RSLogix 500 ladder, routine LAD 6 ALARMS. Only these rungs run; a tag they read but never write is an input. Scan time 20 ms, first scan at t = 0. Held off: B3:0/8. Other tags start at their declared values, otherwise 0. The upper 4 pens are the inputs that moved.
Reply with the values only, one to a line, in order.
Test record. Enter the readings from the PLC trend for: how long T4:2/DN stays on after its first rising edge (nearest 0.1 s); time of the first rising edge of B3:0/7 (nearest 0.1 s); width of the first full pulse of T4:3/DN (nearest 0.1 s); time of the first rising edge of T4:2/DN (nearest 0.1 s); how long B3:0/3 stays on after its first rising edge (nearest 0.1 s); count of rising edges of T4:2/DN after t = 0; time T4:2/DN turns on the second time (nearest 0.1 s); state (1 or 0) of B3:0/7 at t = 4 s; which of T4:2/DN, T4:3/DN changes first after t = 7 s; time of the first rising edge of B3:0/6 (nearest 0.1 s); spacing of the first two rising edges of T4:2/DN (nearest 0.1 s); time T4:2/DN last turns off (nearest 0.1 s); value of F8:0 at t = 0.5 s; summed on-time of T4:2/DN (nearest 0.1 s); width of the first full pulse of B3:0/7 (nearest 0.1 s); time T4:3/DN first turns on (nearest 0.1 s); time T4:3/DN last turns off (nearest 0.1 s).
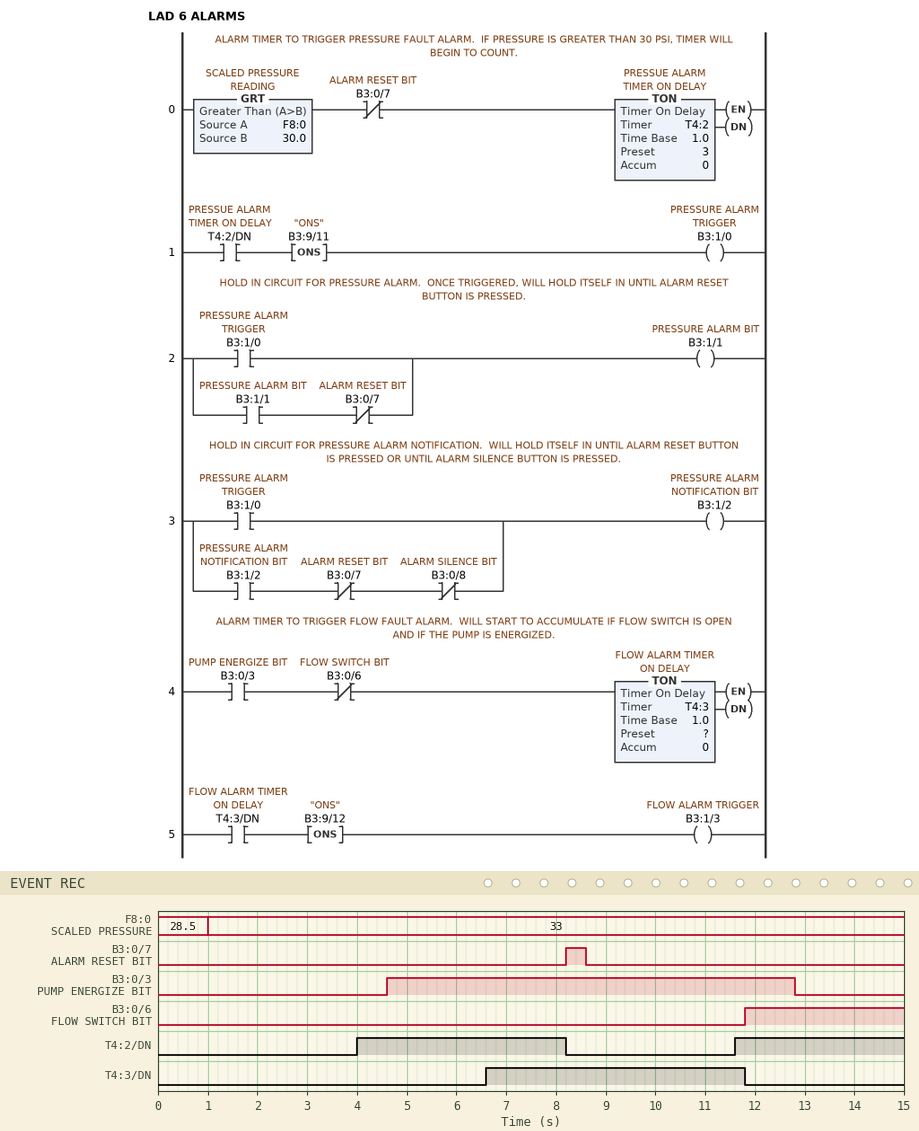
4.2 s
8.2 s
5.2 s
4.0 s
8.2 s
2
11.6 s
0
T4:2/DN
11.8 s
7.6 s
8.2 s
28.5
7.6 s
0.4 s
6.6 s
11.8 s
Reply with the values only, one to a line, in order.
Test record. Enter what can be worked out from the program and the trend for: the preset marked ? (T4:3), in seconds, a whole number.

2 s
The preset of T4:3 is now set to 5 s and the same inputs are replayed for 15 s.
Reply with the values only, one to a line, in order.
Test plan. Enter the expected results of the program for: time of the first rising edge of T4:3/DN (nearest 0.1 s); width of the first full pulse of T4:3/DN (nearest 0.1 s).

9.6 s
2.2 s
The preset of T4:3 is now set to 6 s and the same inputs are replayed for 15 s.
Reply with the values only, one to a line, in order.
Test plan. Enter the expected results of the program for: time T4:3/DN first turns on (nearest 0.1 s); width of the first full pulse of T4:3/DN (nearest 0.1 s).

10.6 s
1.2 s
